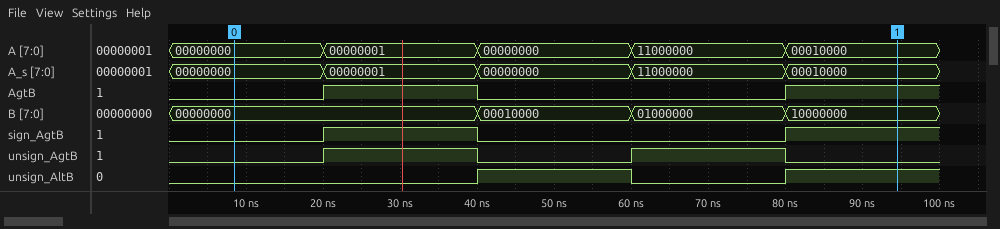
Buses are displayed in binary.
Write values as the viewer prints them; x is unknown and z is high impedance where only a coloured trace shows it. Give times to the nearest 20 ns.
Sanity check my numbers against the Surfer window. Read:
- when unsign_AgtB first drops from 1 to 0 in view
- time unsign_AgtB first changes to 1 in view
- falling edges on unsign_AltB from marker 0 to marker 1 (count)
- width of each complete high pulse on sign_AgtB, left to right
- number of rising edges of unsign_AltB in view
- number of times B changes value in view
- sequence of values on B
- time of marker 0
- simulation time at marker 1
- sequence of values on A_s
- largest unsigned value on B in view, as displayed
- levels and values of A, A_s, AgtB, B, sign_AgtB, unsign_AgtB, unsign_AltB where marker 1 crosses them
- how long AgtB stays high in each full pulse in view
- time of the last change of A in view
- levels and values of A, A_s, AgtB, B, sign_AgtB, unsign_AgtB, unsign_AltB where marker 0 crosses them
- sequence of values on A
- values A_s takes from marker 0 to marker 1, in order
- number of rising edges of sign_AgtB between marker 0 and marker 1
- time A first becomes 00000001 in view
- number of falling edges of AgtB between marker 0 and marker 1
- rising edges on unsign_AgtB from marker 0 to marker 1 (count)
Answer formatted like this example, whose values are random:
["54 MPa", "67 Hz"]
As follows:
["40 ns", "20 ns", "1", "20 ns", "2", "3", "00000000, 00010000, 01000000, 10000000", "0 ns", "100 ns", "00000000, 00000001, 00000000, 11000000, 00010000", "10000000", "A=00010000, A_s=00010000, AgtB=1, B=10000000, sign_AgtB=1, unsign_AgtB=0, unsign_AltB=1", "20 ns", "80 ns", "A=00000000, A_s=00000000, AgtB=0, B=00000000, sign_AgtB=0, unsign_AgtB=0, unsign_AltB=0", "00000000, 00000001, 00000000, 11000000, 00010000", "00000000, 00000001, 00000000, 11000000, 00010000", "2", "20 ns", "1", "2"]
